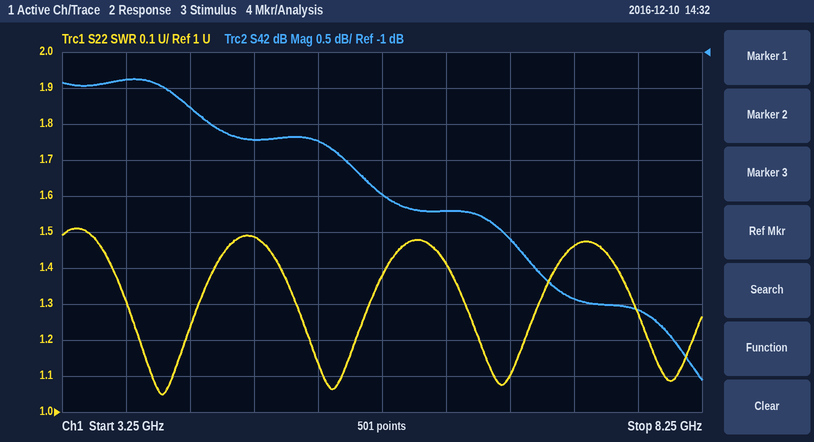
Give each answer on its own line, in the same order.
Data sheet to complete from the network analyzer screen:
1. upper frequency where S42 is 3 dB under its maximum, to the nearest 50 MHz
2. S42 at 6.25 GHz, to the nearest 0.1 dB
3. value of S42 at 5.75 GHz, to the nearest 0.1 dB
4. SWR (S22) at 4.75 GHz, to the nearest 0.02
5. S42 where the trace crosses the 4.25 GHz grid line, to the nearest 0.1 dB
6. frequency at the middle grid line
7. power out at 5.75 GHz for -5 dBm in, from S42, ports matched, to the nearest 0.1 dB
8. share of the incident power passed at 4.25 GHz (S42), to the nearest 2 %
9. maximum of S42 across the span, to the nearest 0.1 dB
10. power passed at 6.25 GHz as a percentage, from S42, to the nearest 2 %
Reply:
7.20 GHz
-3.2 dB
-3.0 dB
1.48
-1.8 dB
5.75 GHz
-8.0 dBm
66 %
-1.4 dB
48 %
